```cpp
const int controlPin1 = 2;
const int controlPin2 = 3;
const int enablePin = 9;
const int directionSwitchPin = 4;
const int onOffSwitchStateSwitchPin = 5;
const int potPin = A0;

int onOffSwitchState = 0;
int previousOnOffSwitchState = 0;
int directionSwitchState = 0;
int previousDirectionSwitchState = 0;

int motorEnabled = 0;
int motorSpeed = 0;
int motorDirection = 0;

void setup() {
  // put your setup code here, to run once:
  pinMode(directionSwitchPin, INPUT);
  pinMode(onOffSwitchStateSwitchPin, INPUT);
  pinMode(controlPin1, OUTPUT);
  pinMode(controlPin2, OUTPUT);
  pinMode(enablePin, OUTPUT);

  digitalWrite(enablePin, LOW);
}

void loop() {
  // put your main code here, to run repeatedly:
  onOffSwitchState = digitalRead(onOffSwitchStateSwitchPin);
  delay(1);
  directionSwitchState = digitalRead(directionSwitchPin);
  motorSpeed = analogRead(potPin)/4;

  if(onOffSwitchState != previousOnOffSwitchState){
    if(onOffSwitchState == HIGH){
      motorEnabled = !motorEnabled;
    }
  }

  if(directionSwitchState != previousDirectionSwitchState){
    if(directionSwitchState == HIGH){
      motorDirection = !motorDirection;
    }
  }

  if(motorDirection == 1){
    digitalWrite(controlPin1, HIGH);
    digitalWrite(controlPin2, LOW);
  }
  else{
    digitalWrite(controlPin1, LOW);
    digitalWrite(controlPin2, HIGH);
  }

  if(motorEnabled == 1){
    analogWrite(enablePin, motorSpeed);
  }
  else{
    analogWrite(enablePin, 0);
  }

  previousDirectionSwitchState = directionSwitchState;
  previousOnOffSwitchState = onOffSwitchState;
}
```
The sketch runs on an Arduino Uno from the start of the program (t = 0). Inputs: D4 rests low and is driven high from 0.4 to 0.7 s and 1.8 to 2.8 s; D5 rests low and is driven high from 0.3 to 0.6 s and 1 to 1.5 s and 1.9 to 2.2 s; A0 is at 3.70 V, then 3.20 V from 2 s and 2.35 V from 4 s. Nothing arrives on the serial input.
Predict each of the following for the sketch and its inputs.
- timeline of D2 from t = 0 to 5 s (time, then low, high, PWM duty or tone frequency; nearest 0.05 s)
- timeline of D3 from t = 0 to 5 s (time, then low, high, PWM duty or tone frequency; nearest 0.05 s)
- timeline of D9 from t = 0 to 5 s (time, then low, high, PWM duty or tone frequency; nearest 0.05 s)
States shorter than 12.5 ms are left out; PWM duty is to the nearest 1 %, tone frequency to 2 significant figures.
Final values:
0 s low; 0.4 s high; 1.8 s low
0 s high; 0.4 s low; 1.8 s high
0 s low; 0.3 s PWM 74 %; 1 s low; 1.9 s PWM 74 %; 2 s PWM 64 %; 4 s PWM 47 %
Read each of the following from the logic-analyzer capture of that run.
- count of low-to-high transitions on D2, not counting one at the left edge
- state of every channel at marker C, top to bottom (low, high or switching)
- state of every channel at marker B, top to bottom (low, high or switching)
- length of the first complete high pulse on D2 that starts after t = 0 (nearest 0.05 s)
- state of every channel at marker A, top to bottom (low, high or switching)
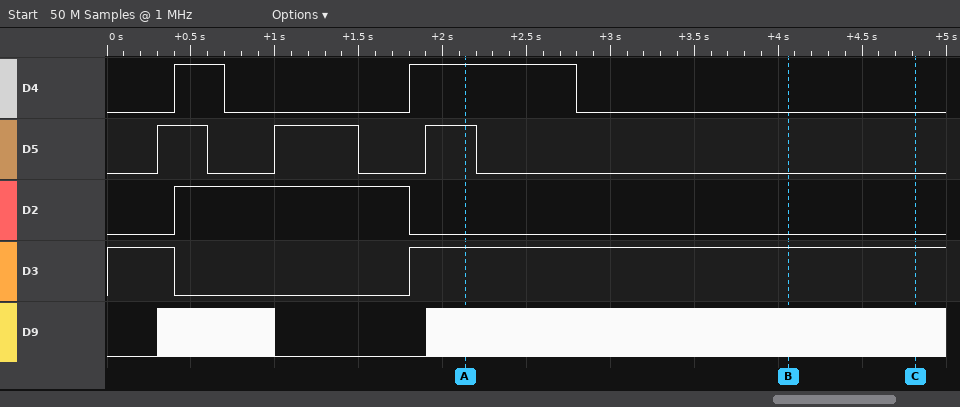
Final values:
1
D4 low, D5 low, D2 low, D3 high, D9 switching
D4 low, D5 low, D2 low, D3 high, D9 switching
1.40 s
D4 high, D5 high, D2 low, D3 high, D9 switching
